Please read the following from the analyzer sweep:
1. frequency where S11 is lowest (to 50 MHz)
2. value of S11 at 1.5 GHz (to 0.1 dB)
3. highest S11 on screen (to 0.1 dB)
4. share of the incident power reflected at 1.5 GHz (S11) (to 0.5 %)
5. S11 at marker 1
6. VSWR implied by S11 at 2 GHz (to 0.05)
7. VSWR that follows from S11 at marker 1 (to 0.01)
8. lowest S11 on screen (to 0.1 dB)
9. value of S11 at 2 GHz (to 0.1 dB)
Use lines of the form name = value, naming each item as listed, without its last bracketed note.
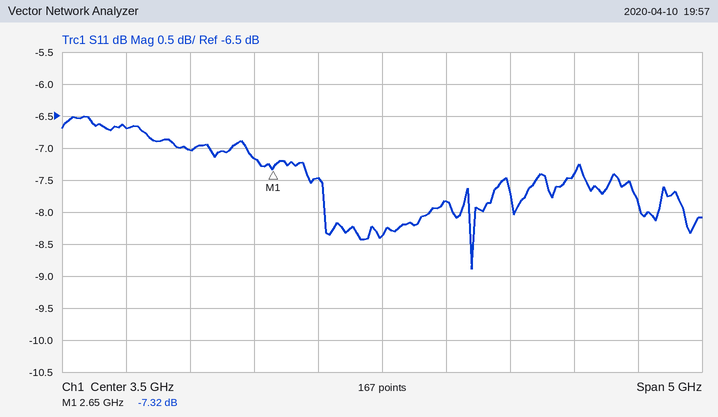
frequency where S11 is lowest = 4.20 GHz
value of S11 at 1.5 GHz = -6.7 dB
highest S11 on screen = -6.5 dB
share of the incident power reflected at 1.5 GHz (S11) = 21.5 %
S11 at marker 1 = -7.32 dB
VSWR implied by S11 at 2 GHz = 2.60
VSWR that follows from S11 at marker 1 = 2.51
lowest S11 on screen = -8.9 dB
value of S11 at 2 GHz = -7.0 dB
